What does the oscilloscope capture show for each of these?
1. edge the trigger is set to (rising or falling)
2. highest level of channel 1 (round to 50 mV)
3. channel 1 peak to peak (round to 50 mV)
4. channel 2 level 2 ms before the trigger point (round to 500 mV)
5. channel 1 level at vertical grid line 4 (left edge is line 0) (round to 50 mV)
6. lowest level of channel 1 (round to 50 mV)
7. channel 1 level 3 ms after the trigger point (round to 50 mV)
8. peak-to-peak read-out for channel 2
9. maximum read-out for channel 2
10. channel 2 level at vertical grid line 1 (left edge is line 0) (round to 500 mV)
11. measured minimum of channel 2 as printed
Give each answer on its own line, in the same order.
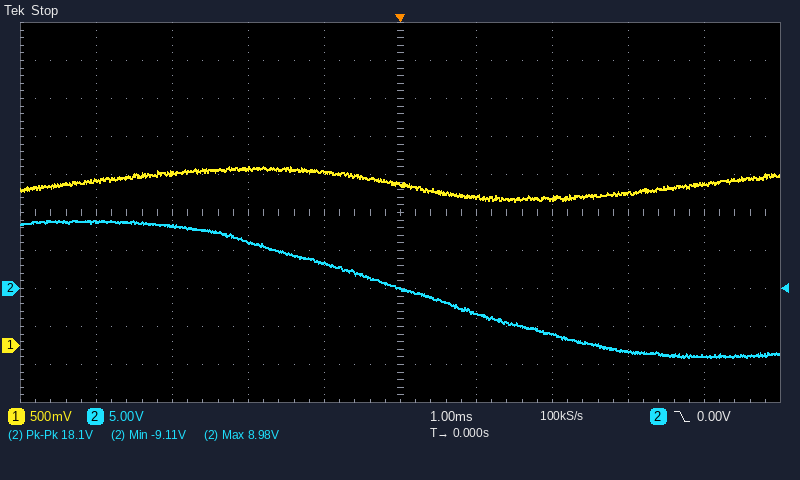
falling
2.35 V
450 mV
6.0 V
2.30 V
1.90 V
2.00 V
18.1 V
8.98 V
9.0 V
-9.11 V
